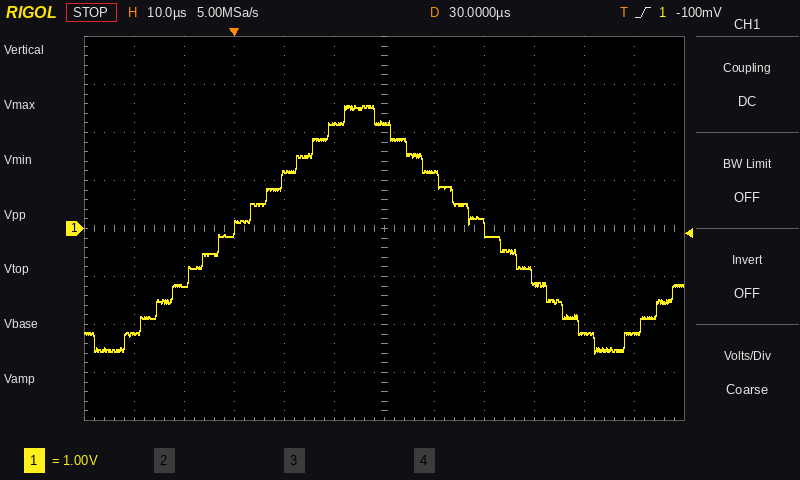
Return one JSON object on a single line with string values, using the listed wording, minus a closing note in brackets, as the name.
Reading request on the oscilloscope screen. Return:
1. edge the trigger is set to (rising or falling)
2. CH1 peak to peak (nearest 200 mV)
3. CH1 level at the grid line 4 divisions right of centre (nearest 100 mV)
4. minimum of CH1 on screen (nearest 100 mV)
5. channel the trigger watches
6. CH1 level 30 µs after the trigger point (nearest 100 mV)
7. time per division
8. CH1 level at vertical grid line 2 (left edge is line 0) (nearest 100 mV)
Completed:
{"edge the trigger is set to": "rising", "CH1 peak to peak": "5.2 V", "CH1 level at the grid line 4 divisions right of centre": "-2.2 V", "minimum of CH1 on screen": "-2.6 V", "channel the trigger watches": "CH1", "CH1 level 30 µs after the trigger point": "2.2 V", "time per division": "10 µs", "CH1 level at vertical grid line 2 (left edge is line 0)": "-1.2 V"}
